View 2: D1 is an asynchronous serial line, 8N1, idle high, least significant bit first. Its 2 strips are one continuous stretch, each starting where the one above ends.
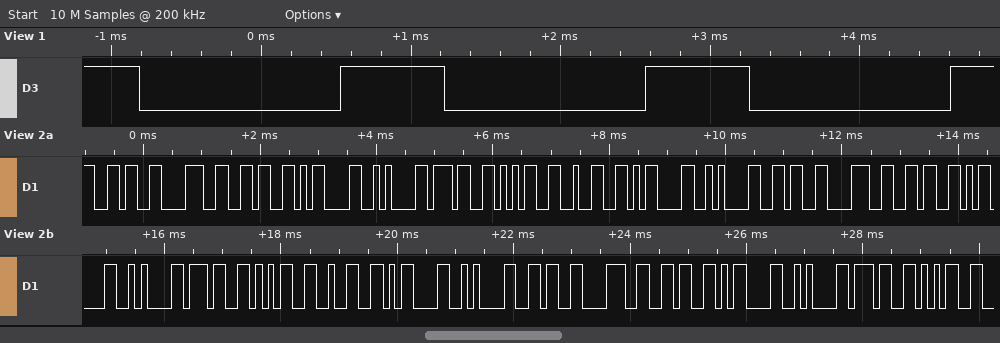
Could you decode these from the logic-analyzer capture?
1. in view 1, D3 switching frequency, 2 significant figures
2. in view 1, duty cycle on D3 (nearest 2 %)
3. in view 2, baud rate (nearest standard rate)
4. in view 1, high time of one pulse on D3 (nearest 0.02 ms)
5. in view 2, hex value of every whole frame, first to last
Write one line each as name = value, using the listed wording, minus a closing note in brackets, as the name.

in view 1, D3 switching frequency, 2 significant figures = 490 Hz
in view 1, duty cycle on D3 = 34 %
in view 2, baud rate = 9600 baud
in view 1, high time of one pulse on D3 = 0.70 ms
in view 2, hex value of every whole frame, first to last = 0x36 0x38 0x36 0x0D 0x0A 0x37 0x35 0x32 0x0D 0x0A 0x36 0x38 0x36 0x0D 0x0A 0x37 0x35 0x32 0x0D 0x0A 0x36 0x38 0x36 0x0D 0x0A 0x37 0x35
